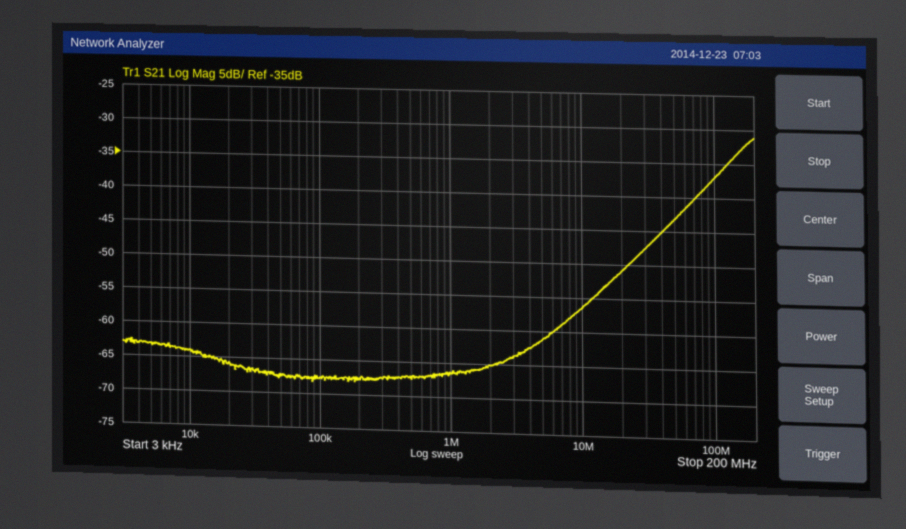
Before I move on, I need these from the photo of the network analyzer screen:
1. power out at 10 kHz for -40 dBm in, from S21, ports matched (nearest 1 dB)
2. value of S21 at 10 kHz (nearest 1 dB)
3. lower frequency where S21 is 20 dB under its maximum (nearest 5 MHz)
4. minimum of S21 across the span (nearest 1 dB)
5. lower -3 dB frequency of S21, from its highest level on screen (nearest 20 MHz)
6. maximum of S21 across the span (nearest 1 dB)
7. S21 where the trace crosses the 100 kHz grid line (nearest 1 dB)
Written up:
-104 dBm
-64 dB
20 MHz
-68 dB
140 MHz
-31 dB
-68 dB
